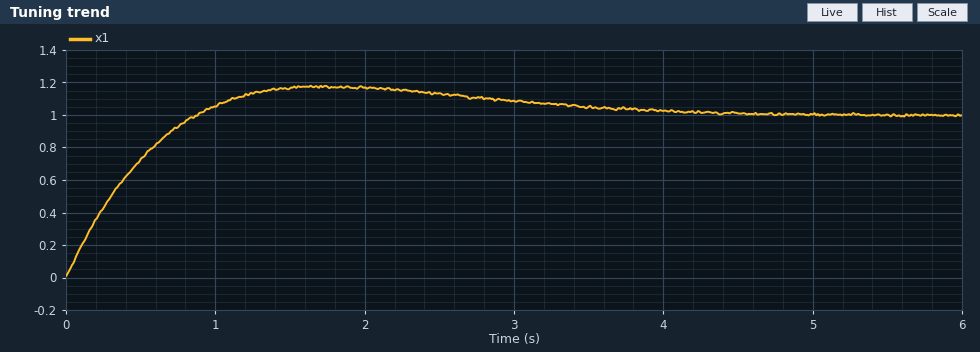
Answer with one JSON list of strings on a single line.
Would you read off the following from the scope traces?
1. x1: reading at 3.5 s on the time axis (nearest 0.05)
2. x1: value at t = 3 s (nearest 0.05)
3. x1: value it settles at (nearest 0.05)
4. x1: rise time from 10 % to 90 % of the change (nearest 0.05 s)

["1.05", "1.10", "1.00", "0.65 s"]
